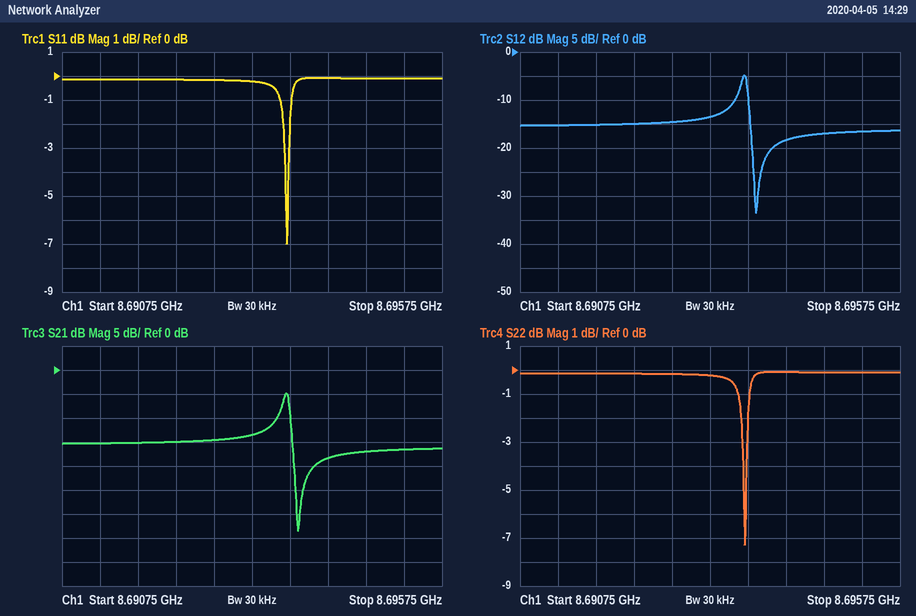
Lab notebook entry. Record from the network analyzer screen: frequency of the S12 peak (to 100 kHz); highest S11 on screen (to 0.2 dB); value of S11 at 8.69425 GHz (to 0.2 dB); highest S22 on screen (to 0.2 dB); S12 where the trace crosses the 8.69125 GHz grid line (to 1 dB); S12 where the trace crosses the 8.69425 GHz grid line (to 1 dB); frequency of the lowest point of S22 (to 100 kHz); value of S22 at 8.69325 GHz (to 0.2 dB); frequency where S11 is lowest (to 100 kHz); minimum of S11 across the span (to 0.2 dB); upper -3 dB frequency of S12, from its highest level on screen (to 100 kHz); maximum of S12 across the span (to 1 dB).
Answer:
8.6937 GHz
0.0 dB
0.0 dB
0.0 dB
-15 dB
-18 dB
8.6937 GHz
-0.2 dB
8.6937 GHz
-7.0 dB
8.6937 GHz
-5 dB
